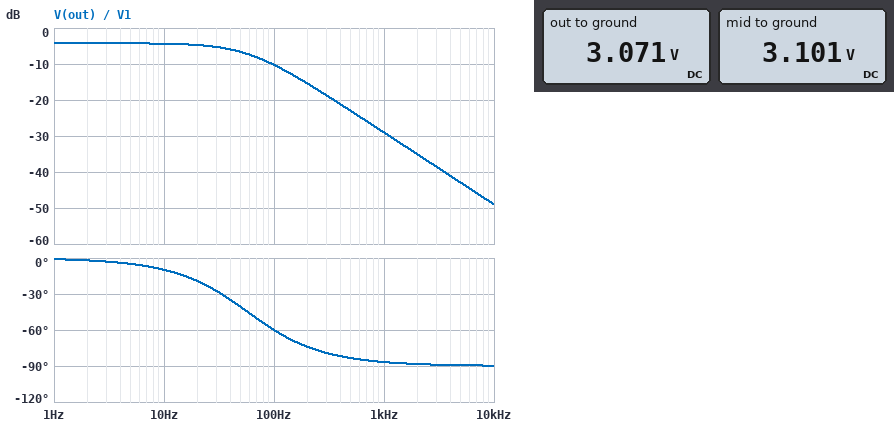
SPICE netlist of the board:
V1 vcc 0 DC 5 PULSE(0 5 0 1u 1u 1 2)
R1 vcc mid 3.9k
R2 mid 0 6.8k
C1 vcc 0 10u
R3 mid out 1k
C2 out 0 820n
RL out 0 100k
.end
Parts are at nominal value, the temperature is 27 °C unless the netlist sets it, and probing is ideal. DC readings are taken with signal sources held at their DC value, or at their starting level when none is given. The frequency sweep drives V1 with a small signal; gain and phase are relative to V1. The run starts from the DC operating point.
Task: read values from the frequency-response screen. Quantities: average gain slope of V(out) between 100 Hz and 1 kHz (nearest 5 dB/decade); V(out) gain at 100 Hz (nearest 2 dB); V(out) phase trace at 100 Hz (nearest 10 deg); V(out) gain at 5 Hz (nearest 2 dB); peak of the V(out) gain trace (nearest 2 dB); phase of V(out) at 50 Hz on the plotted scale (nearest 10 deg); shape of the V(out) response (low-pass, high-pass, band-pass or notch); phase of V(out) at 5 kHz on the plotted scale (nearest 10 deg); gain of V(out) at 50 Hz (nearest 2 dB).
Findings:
-20 dB/decade
-10 dB
-60 deg
-4 dB
-4 dB
-40 deg
low-pass
-90 deg
-6 dB
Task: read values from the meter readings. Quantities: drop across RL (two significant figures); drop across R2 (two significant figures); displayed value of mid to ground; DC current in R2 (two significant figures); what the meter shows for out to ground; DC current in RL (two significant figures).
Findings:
3.1 V
3.1 V
3.101 V
460 µA
3.071 V
31 µA
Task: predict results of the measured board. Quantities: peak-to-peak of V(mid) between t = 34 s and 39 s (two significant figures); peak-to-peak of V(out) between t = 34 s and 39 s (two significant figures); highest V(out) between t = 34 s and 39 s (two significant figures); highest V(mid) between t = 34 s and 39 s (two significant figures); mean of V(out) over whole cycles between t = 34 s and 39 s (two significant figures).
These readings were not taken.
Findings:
3.1 V
3.1 V
3.1 V
3.1 V
1.5 V
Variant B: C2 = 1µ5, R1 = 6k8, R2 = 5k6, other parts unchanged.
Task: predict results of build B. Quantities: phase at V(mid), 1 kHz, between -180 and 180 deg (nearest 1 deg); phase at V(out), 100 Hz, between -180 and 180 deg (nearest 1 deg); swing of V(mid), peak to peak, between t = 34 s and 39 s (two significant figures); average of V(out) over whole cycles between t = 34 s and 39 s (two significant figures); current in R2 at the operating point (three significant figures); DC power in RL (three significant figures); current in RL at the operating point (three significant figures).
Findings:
-5 deg
-75 deg
2.2 V
1.1 V
391 µA
47.1 µW
21.7 µA
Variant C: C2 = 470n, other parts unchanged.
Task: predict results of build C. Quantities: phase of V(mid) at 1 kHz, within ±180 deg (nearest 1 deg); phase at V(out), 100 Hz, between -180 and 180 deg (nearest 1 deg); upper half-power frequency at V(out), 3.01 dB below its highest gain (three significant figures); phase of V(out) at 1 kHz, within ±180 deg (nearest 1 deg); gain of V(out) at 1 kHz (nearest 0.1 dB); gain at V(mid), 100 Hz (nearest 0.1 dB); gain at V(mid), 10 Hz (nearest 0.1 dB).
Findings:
-13 deg
-45 deg
101 Hz
-84 deg
-24.2 dB
-6.8 dB
-4.2 dB
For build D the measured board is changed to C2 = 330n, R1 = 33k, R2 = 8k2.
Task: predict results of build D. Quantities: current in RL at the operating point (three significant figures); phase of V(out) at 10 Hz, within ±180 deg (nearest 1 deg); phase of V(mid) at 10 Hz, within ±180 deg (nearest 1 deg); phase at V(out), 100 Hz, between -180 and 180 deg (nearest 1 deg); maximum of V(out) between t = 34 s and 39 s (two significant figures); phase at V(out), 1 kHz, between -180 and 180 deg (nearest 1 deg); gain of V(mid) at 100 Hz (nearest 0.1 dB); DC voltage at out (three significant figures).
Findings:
9.25 µA
-8 deg
-7 deg
-56 deg
930 mV
-86 deg
-19.3 dB
925 mV
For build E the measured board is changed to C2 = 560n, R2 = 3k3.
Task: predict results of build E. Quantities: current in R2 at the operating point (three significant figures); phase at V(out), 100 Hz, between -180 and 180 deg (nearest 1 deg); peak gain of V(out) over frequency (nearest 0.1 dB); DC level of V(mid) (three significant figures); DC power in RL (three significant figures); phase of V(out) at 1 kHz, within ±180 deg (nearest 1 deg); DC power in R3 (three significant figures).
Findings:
682 µA
-44 deg
-7.0 dB
2.25 V
49.7 µW
-84 deg
497 nW
